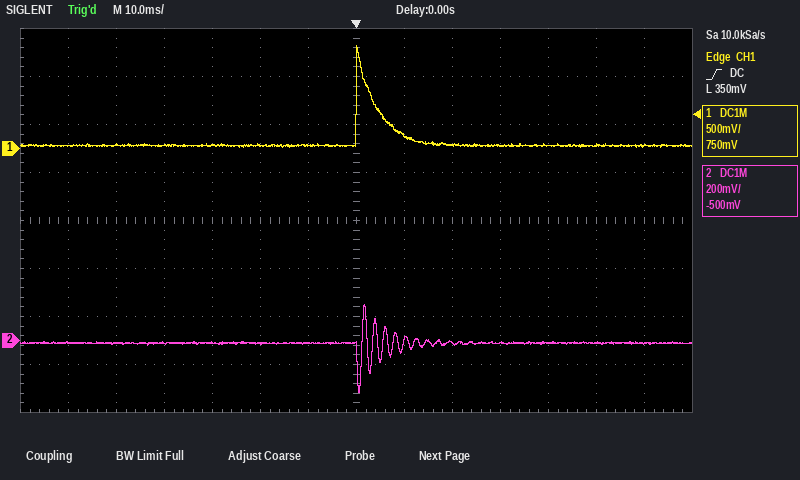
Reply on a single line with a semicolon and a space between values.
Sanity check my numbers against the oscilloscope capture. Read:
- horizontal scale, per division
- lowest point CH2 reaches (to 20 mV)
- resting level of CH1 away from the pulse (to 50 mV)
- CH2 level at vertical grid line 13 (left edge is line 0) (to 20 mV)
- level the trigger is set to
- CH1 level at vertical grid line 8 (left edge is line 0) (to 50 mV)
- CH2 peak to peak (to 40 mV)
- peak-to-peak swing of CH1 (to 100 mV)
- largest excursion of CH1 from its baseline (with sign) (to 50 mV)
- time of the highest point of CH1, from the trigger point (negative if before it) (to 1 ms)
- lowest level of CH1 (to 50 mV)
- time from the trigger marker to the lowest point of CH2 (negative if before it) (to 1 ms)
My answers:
10 ms; -220 mV; 50 mV; -20 mV; 350 mV; 150 mV; 360 mV; 1.10 V; +1.05 V; 0 ms; 0 mV; +1 ms
